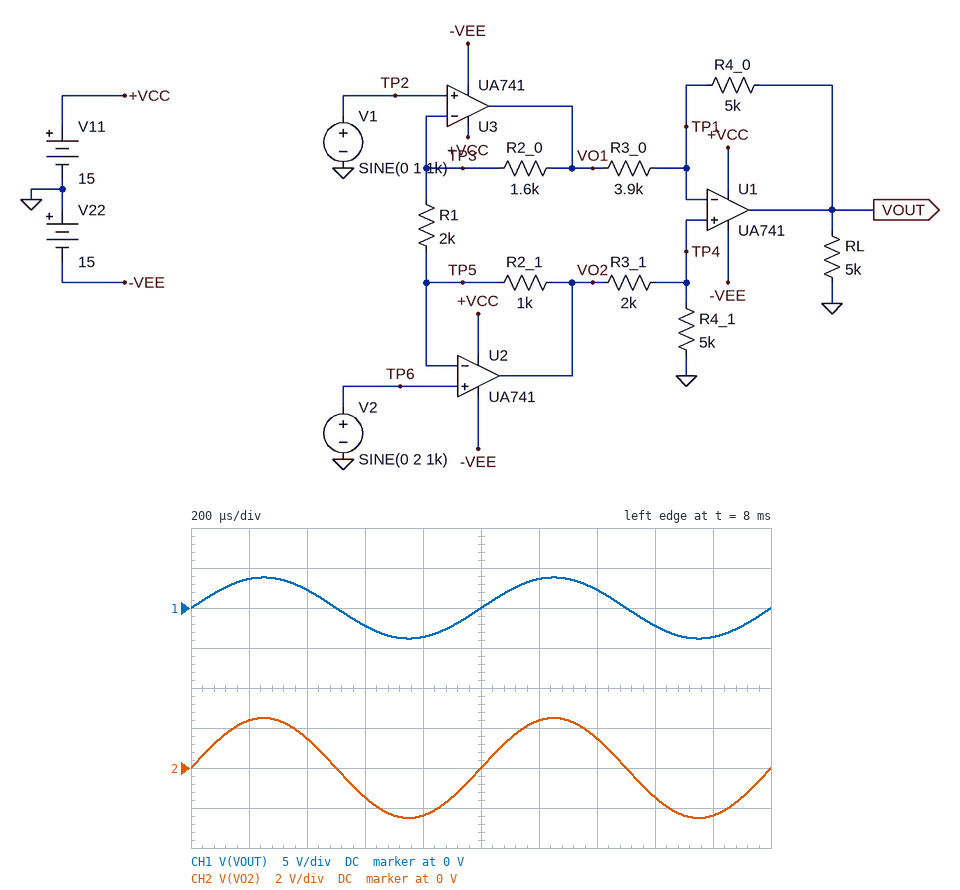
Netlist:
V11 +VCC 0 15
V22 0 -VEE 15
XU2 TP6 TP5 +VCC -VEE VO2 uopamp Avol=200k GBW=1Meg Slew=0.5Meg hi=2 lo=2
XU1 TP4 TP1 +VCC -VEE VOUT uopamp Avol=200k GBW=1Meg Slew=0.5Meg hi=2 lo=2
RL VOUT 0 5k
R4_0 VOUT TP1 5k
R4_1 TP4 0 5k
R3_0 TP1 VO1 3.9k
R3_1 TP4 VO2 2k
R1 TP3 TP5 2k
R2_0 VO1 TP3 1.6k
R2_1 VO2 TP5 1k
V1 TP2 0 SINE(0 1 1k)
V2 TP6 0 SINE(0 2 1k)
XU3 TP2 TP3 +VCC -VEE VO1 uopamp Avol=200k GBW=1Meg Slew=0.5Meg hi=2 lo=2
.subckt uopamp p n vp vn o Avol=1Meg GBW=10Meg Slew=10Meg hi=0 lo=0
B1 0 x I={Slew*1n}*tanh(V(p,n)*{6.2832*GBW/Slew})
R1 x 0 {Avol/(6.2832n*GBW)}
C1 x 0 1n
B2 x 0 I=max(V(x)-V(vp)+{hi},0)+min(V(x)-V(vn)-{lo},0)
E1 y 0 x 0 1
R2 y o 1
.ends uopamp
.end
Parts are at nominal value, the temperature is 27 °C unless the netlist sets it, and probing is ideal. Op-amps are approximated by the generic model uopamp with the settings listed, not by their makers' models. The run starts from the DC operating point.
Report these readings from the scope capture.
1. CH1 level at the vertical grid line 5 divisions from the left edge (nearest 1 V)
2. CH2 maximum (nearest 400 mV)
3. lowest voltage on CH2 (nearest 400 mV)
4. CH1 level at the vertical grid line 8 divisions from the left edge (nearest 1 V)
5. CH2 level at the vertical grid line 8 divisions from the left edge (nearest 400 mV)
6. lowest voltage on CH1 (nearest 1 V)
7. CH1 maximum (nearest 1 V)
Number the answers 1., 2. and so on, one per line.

1. 0 V
2. 2.4 V
3. -2.4 V
4. -2 V
5. -1.6 V
6. -4 V
7. 4 V
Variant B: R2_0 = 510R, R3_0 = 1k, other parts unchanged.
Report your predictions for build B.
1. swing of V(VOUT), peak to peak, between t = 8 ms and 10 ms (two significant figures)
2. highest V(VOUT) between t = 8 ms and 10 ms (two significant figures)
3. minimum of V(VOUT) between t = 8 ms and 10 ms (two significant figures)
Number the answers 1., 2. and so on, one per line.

1. 14 V
2. 7.0 V
3. -7.0 V
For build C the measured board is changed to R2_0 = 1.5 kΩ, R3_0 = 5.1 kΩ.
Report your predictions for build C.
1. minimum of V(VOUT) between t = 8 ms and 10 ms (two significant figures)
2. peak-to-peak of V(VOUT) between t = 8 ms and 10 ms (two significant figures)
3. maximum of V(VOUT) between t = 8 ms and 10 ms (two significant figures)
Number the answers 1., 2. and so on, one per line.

1. -3.3 V
2. 6.6 V
3. 3.3 V
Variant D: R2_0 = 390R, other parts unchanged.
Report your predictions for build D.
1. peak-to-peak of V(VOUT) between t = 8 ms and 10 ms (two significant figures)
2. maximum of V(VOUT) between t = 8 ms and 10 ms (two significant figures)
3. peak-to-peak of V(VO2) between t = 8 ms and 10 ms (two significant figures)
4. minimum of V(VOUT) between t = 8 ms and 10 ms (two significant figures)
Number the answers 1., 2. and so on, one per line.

1. 6.1 V
2. 3.0 V
3. 5.0 V
4. -3.0 V
